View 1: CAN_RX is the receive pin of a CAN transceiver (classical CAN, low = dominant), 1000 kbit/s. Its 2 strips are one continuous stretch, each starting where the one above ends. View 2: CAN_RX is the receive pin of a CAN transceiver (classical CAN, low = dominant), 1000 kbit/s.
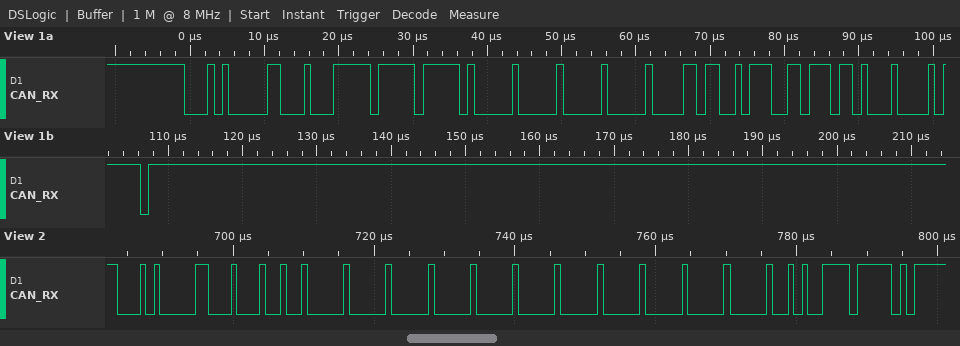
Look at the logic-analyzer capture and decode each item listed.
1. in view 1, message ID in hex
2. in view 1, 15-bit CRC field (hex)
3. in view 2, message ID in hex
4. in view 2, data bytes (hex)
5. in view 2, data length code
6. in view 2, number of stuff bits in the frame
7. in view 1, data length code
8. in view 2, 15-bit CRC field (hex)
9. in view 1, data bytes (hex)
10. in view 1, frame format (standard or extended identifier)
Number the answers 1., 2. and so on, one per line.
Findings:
1. 0x141
2. 0x442F
3. 0x141
4. 92 00 00 00 00 00 00 00
5. 8
6. 13
7. 8
8. 0x53DF
9. FF FF 00 00 00 D9 73 76
10. standard
